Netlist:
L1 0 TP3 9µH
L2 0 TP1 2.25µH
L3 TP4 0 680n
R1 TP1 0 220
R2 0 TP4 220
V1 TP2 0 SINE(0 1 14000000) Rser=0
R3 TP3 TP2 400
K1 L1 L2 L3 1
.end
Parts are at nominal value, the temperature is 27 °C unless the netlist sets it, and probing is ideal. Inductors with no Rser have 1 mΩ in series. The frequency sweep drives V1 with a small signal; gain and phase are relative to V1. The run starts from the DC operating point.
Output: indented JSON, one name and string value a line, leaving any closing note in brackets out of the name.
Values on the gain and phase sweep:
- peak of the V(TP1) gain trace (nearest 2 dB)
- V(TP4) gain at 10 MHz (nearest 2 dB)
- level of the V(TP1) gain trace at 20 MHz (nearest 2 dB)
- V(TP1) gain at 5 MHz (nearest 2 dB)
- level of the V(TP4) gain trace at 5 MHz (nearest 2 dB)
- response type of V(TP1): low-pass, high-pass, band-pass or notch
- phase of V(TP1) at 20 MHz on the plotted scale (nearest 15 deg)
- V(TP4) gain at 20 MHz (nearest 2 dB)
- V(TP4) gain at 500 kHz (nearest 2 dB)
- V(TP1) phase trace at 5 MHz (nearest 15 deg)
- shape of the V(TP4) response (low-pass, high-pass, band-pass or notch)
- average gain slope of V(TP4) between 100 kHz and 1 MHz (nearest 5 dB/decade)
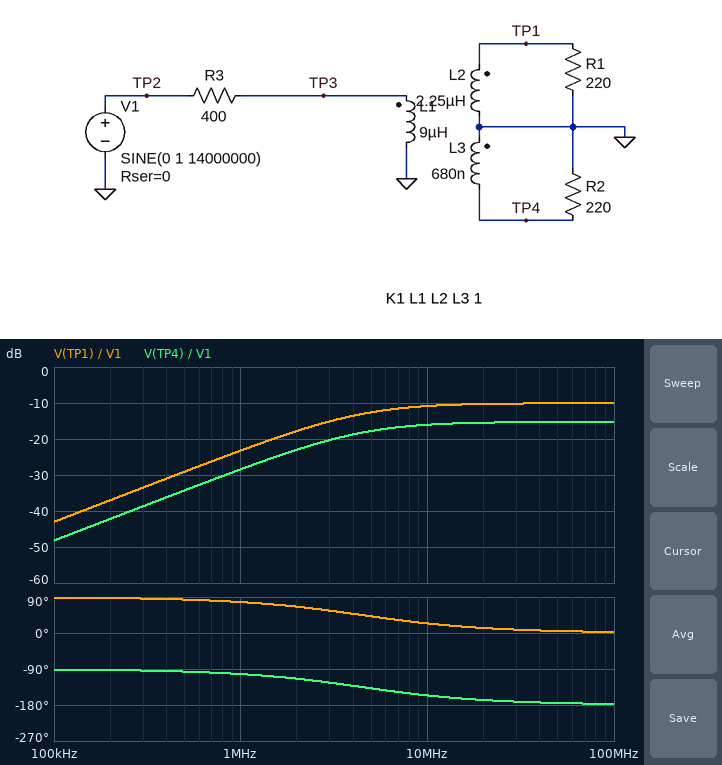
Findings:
{
  "peak of the V(TP1) gain trace": "-10 dB",
  "V(TP4) gain at 10 MHz": "-16 dB",
  "level of the V(TP1) gain trace at 20 MHz": "-10 dB",
  "V(TP1) gain at 5 MHz": "-12 dB",
  "level of the V(TP4) gain trace at 5 MHz": "-18 dB",
  "response type of V(TP1): low-pass, high-pass, band-pass or notch": "high-pass",
  "phase of V(TP1) at 20 MHz on the plotted scale": "15 deg",
  "V(TP4) gain at 20 MHz": "-16 dB",
  "V(TP4) gain at 500 kHz": "-34 dB",
  "V(TP1) phase trace at 5 MHz": "45 deg",
  "shape of the V(TP4) response": "high-pass",
  "average gain slope of V(TP4) between 100 kHz and 1 MHz": "20 dB/decade"
}
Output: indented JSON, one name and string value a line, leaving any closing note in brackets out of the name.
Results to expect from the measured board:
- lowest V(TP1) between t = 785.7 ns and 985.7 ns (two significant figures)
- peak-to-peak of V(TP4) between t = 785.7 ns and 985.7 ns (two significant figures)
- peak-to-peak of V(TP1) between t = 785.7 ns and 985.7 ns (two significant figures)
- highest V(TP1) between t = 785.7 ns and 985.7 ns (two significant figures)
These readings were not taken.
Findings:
{
  "lowest V(TP1) between t = 785.7 ns and 985.7 ns": "-300 mV",
  "peak-to-peak of V(TP4) between t = 785.7 ns and 985.7 ns": "330 mV",
  "peak-to-peak of V(TP1) between t = 785.7 ns and 985.7 ns": "600 mV",
  "highest V(TP1) between t = 785.7 ns and 985.7 ns": "300 mV"
}
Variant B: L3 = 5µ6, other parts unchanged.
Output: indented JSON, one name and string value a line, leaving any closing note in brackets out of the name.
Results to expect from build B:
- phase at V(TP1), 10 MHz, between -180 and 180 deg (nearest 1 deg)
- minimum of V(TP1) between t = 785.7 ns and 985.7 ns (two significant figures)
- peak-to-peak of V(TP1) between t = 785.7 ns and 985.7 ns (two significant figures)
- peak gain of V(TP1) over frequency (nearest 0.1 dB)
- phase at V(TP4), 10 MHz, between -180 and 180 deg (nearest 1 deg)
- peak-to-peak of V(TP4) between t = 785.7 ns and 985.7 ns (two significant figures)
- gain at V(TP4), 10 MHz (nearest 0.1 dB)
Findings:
{
  "phase at V(TP1), 10 MHz, between -180 and 180 deg": "15 deg",
  "minimum of V(TP1) between t = 785.7 ns and 985.7 ns": "-190 mV",
  "peak-to-peak of V(TP1) between t = 785.7 ns and 985.7 ns": "380 mV",
  "peak gain of V(TP1) over frequency": "-14.3 dB",
  "phase at V(TP4), 10 MHz, between -180 and 180 deg": "-165 deg",
  "peak-to-peak of V(TP4) between t = 785.7 ns and 985.7 ns": "600 mV",
  "gain at V(TP4), 10 MHz": "-10.6 dB"
}
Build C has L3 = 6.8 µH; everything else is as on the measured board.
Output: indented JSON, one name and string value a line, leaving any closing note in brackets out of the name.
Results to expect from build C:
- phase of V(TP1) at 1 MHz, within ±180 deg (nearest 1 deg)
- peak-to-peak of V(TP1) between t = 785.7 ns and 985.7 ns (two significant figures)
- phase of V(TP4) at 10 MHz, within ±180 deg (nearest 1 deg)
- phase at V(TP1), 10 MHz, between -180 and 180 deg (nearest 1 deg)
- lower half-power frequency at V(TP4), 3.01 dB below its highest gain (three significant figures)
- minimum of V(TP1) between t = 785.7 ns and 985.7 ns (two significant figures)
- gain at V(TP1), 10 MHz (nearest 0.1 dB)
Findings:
{
  "phase of V(TP1) at 1 MHz, within ±180 deg": "68 deg",
  "peak-to-peak of V(TP1) between t = 785.7 ns and 985.7 ns": "350 mV",
  "phase of V(TP4) at 10 MHz, within ±180 deg": "-166 deg",
  "phase at V(TP1), 10 MHz, between -180 and 180 deg": "14 deg",
  "lower half-power frequency at V(TP4), 3.01 dB below its highest gain": "2.50 MHz",
  "minimum of V(TP1) between t = 785.7 ns and 985.7 ns": "-170 mV",
  "gain at V(TP1), 10 MHz": "-15.3 dB"
}
